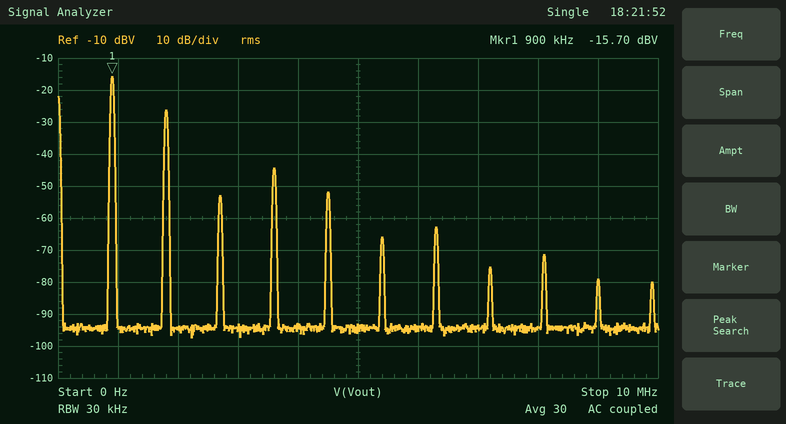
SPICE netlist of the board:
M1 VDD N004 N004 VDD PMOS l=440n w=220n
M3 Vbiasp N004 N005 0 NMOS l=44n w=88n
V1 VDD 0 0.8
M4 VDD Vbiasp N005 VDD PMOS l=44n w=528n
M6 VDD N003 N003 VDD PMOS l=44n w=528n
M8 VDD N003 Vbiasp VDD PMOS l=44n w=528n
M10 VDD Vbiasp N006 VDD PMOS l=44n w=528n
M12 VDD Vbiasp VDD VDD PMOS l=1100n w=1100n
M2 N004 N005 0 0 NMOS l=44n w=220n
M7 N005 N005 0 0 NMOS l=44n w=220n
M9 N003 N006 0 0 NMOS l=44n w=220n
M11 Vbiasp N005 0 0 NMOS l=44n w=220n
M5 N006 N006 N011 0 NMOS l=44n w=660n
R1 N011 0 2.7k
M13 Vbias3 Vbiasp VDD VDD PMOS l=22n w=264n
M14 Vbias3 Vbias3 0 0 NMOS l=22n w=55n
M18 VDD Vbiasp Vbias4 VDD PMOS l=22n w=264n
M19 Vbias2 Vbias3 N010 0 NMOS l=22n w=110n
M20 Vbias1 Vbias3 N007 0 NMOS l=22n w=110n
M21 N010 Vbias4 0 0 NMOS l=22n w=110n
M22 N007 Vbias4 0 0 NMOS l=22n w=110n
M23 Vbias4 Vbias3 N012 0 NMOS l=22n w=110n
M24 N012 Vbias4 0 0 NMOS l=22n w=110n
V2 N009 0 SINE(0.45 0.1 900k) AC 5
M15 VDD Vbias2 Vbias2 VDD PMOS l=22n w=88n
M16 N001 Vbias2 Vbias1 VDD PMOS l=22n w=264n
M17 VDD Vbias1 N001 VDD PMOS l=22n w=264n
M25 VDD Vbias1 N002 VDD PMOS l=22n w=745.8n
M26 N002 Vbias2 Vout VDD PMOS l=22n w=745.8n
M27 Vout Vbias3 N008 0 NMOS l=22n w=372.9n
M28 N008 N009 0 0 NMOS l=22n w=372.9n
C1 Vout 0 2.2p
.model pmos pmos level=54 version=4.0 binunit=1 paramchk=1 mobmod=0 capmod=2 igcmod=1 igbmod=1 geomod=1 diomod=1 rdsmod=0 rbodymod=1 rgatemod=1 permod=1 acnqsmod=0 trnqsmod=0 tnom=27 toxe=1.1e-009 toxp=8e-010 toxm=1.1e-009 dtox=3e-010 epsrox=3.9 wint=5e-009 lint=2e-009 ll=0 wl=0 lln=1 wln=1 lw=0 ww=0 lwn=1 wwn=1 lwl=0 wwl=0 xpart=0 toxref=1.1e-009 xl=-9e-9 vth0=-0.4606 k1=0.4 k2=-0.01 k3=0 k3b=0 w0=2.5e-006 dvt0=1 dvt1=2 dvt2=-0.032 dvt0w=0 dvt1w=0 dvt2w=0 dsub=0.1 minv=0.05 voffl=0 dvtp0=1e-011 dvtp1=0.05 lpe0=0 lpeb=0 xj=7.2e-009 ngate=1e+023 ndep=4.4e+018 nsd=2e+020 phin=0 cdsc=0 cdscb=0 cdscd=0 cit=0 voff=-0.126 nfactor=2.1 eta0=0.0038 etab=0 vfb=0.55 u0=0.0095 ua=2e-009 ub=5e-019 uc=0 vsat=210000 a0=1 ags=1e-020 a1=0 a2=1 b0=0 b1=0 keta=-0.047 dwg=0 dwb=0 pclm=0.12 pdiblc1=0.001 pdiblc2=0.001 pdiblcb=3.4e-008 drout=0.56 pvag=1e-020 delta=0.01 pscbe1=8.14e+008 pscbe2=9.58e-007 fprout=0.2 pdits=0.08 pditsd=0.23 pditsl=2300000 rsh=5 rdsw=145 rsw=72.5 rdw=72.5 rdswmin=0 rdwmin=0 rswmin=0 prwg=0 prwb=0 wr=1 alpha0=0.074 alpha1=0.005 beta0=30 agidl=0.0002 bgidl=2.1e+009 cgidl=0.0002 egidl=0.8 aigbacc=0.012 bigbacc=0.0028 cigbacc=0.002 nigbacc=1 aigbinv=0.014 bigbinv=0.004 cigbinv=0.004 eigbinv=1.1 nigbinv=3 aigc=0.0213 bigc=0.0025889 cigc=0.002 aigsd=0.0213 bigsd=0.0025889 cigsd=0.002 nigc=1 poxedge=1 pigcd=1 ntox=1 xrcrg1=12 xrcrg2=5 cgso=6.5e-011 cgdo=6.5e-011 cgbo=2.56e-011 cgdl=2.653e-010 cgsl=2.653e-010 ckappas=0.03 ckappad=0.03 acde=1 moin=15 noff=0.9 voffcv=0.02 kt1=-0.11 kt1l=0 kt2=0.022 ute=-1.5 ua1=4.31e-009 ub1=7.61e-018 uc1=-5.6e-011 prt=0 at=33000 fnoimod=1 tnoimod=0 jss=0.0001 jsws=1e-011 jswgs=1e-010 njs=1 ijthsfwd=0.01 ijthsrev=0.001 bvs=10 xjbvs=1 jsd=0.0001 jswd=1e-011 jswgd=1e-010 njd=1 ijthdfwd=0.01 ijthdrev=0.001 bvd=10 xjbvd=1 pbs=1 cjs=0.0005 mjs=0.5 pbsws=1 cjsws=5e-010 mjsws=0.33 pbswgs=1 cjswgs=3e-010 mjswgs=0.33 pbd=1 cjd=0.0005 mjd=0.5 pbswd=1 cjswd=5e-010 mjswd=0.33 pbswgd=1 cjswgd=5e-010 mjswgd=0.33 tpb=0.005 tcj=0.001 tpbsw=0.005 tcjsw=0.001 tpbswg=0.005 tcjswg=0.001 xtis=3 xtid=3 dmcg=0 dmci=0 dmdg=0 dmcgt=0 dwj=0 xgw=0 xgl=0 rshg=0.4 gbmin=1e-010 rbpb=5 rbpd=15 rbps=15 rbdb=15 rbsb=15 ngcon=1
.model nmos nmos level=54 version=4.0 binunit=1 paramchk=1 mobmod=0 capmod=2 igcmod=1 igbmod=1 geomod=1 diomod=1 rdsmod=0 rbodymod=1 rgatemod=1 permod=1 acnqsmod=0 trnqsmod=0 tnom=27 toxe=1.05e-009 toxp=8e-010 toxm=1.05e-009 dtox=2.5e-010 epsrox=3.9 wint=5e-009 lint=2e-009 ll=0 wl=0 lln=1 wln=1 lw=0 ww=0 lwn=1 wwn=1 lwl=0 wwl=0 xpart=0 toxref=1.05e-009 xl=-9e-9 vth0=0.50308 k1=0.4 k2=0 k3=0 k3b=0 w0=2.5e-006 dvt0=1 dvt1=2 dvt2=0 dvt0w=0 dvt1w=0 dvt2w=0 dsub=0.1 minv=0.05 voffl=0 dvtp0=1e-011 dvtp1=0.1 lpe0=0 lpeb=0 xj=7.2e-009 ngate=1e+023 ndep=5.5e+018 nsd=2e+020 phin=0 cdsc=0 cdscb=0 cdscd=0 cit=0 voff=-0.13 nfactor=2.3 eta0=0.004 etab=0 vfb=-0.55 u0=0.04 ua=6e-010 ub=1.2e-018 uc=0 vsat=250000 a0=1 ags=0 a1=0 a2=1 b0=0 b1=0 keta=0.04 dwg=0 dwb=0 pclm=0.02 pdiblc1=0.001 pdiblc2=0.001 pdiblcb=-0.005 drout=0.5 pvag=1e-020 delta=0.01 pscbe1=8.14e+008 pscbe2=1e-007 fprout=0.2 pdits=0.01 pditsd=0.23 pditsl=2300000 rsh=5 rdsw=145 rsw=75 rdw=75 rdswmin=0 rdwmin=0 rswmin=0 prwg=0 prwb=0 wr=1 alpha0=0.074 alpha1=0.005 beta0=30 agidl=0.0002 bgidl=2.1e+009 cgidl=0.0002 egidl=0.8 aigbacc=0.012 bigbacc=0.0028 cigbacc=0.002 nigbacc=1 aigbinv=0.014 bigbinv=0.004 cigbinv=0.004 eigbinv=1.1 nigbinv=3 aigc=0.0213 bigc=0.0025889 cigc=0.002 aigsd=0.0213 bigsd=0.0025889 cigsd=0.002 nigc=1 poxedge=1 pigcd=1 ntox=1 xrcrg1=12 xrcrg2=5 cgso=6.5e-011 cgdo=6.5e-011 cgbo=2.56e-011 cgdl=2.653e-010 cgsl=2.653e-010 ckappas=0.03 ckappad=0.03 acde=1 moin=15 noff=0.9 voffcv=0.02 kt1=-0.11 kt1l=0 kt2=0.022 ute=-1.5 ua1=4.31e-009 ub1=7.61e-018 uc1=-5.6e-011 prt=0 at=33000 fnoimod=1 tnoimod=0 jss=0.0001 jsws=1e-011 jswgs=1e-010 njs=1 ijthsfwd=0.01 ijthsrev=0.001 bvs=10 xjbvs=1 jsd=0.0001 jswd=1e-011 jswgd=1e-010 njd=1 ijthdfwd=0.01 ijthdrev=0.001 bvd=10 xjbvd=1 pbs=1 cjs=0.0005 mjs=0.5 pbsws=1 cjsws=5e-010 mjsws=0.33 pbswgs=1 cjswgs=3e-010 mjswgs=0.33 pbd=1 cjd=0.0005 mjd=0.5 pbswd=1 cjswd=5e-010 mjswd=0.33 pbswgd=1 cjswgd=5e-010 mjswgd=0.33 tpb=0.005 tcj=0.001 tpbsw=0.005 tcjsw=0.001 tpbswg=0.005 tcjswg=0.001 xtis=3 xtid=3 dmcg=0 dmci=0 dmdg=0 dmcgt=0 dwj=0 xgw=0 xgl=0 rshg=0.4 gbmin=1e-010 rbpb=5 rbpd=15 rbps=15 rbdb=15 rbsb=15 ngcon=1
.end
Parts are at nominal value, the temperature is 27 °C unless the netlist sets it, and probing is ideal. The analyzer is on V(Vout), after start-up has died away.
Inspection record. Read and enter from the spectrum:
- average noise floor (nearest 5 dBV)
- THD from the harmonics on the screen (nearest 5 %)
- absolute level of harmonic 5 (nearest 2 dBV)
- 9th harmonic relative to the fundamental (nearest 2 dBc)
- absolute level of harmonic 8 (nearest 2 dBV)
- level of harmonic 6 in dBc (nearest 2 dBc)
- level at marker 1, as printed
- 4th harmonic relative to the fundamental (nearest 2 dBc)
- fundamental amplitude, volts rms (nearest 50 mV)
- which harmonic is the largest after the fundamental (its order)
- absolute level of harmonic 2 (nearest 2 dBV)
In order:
-95 dBV
30 %
-52 dBV
-56 dBc
-76 dBV
-50 dBc
-15.70 dBV
-28 dBc
150 mV
2
-26 dBV
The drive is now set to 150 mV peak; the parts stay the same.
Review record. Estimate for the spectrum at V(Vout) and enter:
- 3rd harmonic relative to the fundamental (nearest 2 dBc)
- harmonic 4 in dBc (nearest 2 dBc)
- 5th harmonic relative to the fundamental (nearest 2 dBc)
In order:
-24 dBc
-22 dBc
-34 dBc
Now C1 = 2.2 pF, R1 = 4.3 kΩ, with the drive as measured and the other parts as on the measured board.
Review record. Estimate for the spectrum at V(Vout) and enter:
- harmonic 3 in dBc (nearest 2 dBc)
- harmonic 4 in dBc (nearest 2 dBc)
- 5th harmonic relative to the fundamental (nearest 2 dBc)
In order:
-32 dBc
-26 dBc
-42 dBc
